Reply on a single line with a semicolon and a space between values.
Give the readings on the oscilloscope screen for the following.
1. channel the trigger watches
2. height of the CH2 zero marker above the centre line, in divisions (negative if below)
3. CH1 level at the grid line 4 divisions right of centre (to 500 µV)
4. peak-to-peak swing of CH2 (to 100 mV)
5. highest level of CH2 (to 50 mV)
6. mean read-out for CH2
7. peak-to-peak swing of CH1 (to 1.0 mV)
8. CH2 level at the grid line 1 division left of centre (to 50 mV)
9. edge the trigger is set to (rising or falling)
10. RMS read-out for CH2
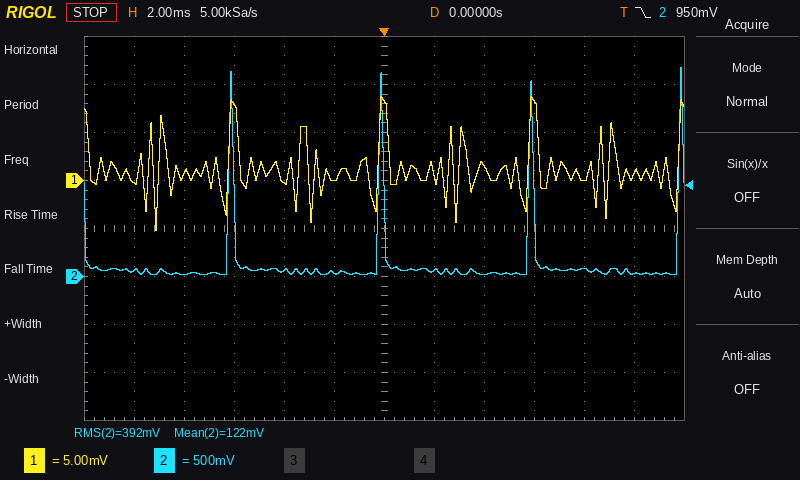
CH2; -1.0 div; 0.0 mV; 2.20 V; 2.20 V; 122 mV; 14.0 mV; 50 mV; falling; 392 mV
